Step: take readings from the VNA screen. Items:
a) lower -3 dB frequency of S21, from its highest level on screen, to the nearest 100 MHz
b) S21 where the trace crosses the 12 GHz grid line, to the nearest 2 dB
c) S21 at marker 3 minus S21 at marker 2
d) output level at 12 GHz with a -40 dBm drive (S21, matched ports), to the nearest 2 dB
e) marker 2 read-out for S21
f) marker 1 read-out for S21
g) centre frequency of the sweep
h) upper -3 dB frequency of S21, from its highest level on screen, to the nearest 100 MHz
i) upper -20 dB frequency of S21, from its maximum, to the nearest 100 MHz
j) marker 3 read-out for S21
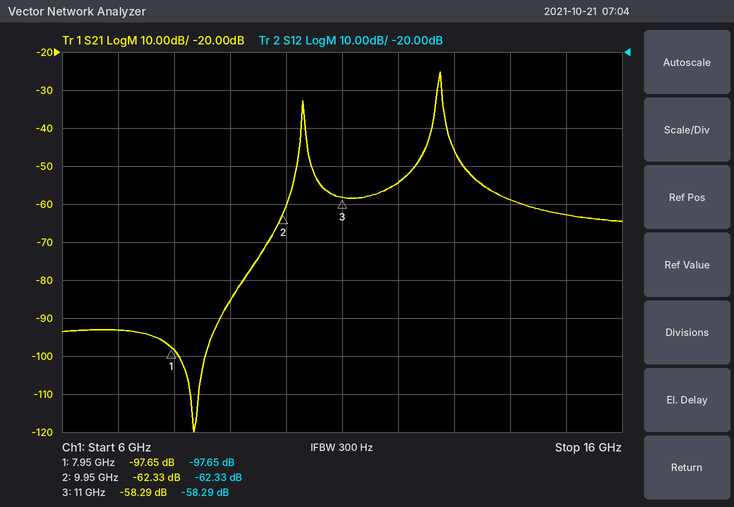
12.7 GHz
-54 dB
4.04 dB
-94 dBm
-62.33 dB
-97.65 dB
11 GHz
12.8 GHz
13.0 GHz
-58.29 dB
